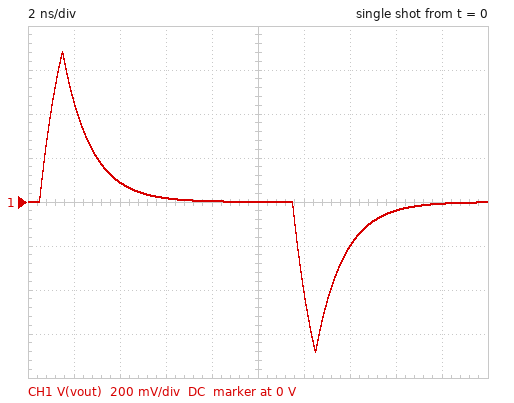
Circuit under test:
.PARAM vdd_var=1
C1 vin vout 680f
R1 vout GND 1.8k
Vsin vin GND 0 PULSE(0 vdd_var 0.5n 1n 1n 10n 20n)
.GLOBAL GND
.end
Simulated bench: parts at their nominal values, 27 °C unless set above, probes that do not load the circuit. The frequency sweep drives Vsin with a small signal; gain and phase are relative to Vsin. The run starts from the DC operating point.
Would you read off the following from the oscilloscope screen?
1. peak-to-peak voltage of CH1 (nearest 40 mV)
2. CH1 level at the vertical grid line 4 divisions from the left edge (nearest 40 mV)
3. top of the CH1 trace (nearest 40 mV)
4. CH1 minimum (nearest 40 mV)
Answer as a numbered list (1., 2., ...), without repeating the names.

1. 1.36 V
2. 0 V
3. 680 mV
4. -680 mV
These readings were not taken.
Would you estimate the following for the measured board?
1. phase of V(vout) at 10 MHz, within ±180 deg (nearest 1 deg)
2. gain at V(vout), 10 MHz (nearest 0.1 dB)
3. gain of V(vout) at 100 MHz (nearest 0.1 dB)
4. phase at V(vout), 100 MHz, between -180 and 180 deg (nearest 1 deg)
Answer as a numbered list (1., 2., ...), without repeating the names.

1. 86 deg
2. -22.3 dB
3. -4.3 dB
4. 52 deg
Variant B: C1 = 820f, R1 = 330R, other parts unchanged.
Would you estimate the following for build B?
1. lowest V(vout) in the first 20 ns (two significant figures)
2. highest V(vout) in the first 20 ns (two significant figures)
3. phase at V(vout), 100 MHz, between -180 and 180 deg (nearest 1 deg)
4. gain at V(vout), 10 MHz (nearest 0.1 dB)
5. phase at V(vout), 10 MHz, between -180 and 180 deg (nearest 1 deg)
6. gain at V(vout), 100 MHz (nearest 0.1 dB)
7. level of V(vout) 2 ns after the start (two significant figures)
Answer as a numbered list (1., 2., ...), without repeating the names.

1. -260 mV
2. 260 mV
3. 80 deg
4. -35.4 dB
5. 89 deg
6. -15.5 dB
7. 42 mV
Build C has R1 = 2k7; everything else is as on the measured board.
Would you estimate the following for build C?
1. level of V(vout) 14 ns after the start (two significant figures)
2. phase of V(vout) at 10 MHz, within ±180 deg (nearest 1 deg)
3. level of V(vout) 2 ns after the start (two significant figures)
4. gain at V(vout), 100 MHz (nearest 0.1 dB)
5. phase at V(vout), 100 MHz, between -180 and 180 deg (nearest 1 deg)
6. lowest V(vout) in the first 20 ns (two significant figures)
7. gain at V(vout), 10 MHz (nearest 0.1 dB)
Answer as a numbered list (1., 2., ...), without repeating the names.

1. -340 mV
2. 83 deg
3. 590 mV
4. -2.4 dB
5. 41 deg
6. -770 mV
7. -18.8 dB
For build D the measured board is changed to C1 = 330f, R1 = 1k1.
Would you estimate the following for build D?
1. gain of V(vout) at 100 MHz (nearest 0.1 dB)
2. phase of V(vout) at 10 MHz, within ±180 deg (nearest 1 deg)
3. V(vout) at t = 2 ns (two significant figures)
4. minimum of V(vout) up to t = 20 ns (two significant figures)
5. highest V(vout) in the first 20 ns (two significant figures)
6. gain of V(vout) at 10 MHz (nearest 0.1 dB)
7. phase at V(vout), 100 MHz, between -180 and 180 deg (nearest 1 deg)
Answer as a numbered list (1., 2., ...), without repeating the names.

1. -13.1 dB
2. 89 deg
3. 86 mV
4. -340 mV
5. 340 mV
6. -32.8 dB
7. 77 deg
